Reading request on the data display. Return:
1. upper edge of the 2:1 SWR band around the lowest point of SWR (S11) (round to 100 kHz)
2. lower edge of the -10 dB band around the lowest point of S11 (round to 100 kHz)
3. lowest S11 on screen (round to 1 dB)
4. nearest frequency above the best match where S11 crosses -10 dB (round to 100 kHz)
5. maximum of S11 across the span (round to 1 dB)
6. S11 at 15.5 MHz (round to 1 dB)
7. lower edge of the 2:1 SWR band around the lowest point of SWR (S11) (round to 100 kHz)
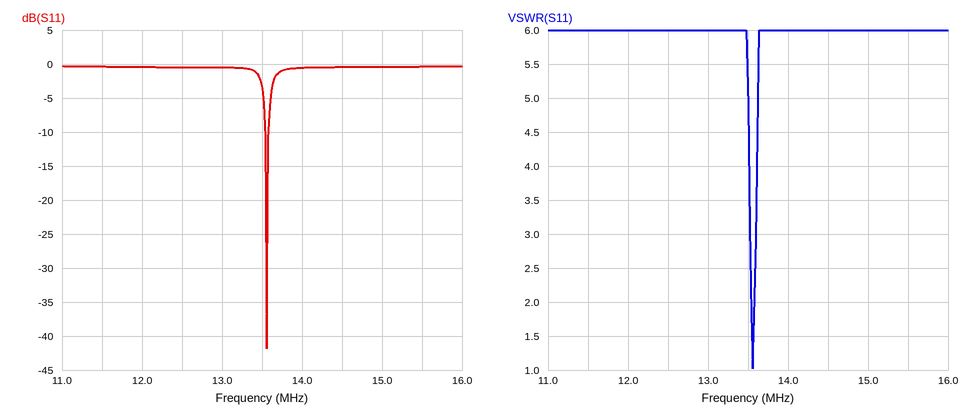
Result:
13.6 MHz
13.5 MHz
-42 dB
13.6 MHz
0 dB
0 dB
13.5 MHz
